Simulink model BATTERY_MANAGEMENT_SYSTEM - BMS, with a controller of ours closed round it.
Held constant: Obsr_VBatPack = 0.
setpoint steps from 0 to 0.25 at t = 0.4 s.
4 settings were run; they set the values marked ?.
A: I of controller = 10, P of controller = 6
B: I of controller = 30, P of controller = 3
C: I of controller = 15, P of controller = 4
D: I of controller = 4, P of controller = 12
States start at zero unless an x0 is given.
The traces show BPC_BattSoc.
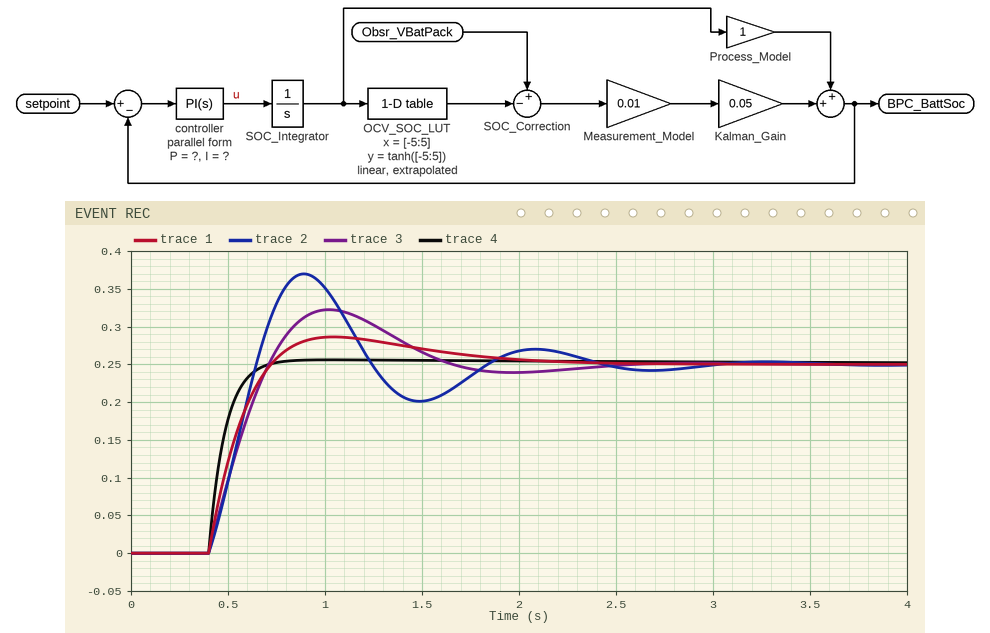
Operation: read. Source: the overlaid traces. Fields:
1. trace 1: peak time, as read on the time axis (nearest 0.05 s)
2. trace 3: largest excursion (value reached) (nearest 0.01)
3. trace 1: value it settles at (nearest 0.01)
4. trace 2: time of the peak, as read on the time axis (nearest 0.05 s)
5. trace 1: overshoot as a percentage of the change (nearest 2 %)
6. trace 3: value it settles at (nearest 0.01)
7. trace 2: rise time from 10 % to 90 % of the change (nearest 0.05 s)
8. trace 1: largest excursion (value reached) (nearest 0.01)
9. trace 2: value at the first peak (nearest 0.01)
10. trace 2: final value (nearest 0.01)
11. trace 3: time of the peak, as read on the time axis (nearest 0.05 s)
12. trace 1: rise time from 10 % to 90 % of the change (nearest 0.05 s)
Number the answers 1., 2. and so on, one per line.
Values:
1. 1.05 s
2. 0.32
3. 0.25
4. 0.90 s
5. 14 %
6. 0.25
7. 0.20 s
8. 0.29
9. 0.37
10. 0.25
11. 1.00 s
12. 0.25 s
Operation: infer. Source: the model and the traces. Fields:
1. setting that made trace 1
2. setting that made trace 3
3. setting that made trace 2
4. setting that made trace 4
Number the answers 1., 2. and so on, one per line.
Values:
1. A
2. C
3. B
4. D
